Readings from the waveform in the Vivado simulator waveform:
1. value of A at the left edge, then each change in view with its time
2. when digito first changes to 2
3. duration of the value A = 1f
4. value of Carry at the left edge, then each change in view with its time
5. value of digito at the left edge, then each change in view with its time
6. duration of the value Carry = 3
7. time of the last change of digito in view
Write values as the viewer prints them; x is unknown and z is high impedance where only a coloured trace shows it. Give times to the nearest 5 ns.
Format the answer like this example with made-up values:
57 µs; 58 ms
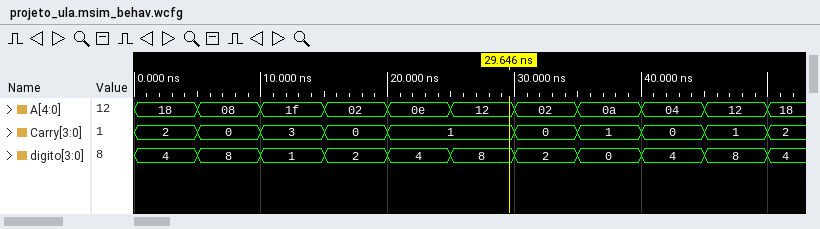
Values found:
18, 08 at 5 ns, 1f at 10 ns, 02 at 15 ns, 0e at 20 ns, 12 at 25 ns, 02 at 30 ns, 0a at 35 ns, 04 at 40 ns, 12 at 45 ns, 18 at 50 ns; 15 ns; 5 ns; 2, 0 at 5 ns, 3 at 10 ns, 0 at 15 ns, 1 at 20 ns, 0 at 30 ns, 1 at 35 ns, 0 at 40 ns, 1 at 45 ns, 2 at 50 ns; 4, 8 at 5 ns, 1 at 10 ns, 2 at 15 ns, 4 at 20 ns, 8 at 25 ns, 2 at 30 ns, 0 at 35 ns, 4 at 40 ns, 8 at 45 ns, 4 at 50 ns; 5 ns; 50 ns
